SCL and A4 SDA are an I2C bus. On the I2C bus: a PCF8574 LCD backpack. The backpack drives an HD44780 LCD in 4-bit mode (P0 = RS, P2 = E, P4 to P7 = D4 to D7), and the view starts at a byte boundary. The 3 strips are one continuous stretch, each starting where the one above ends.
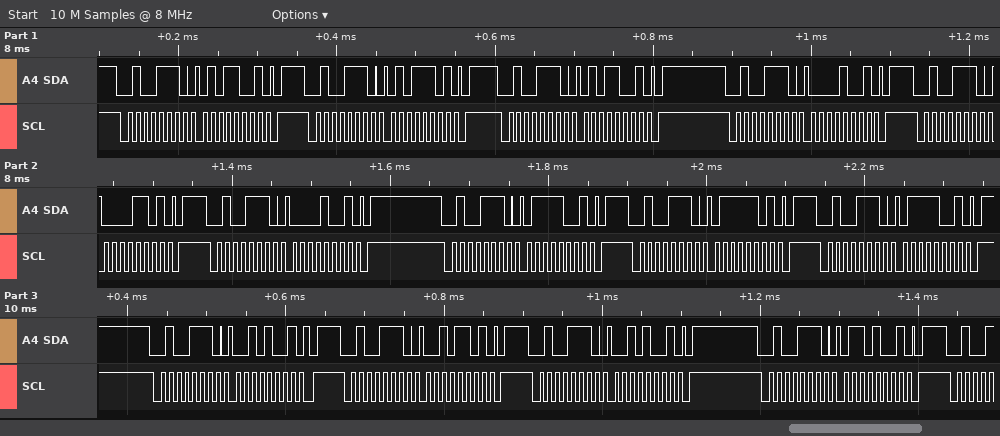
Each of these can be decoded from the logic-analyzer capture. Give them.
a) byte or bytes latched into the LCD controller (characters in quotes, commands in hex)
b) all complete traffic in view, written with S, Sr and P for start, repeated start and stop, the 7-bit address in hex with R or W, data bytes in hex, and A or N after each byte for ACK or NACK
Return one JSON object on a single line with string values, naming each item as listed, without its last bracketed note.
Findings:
{"byte or bytes latched into the LCD controller": "'P' 'r'", "all complete traffic in view, written with S, Sr and P for start, repeated start and stop, the 7-bit address in hex with R or W, data bytes in hex, and A or N after each byte for ACK or NACK": "S 27W A 59 A P S 27W A 5D A P S 27W A 59 A P S 27W A 09 A P S 27W A 0D A P S 27W A 09 A P S 27W A 79 A P S 27W A 7D A P S 27W A 79 A P S 27W A 29 A P S 27W A 2D A P S 27W A 29 A P S 27W A 69 A P"}
